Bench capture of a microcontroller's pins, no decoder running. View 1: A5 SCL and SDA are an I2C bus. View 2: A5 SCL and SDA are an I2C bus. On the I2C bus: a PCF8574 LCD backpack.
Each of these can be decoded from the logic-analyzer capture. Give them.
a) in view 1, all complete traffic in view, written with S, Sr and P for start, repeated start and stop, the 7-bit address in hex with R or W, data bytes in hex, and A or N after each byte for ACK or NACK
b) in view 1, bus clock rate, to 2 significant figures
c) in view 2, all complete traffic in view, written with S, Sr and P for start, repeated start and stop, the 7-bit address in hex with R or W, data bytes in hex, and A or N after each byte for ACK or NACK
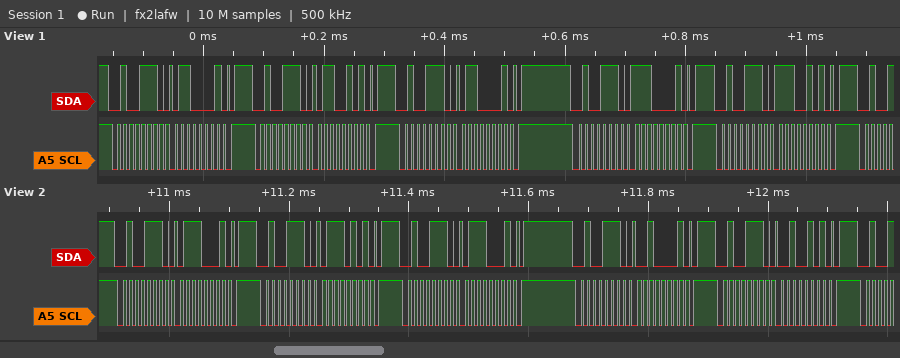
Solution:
S 27W A 61 A P S 27W A 65 A P S 27W A 61 A P S 27W A E1 A P S 27W A E5 A P
100 kHz
S 27W A 71 A P S 27W A 75 A P S 27W A 71 A P S 27W A 21 A P S 27W A 25 A P
